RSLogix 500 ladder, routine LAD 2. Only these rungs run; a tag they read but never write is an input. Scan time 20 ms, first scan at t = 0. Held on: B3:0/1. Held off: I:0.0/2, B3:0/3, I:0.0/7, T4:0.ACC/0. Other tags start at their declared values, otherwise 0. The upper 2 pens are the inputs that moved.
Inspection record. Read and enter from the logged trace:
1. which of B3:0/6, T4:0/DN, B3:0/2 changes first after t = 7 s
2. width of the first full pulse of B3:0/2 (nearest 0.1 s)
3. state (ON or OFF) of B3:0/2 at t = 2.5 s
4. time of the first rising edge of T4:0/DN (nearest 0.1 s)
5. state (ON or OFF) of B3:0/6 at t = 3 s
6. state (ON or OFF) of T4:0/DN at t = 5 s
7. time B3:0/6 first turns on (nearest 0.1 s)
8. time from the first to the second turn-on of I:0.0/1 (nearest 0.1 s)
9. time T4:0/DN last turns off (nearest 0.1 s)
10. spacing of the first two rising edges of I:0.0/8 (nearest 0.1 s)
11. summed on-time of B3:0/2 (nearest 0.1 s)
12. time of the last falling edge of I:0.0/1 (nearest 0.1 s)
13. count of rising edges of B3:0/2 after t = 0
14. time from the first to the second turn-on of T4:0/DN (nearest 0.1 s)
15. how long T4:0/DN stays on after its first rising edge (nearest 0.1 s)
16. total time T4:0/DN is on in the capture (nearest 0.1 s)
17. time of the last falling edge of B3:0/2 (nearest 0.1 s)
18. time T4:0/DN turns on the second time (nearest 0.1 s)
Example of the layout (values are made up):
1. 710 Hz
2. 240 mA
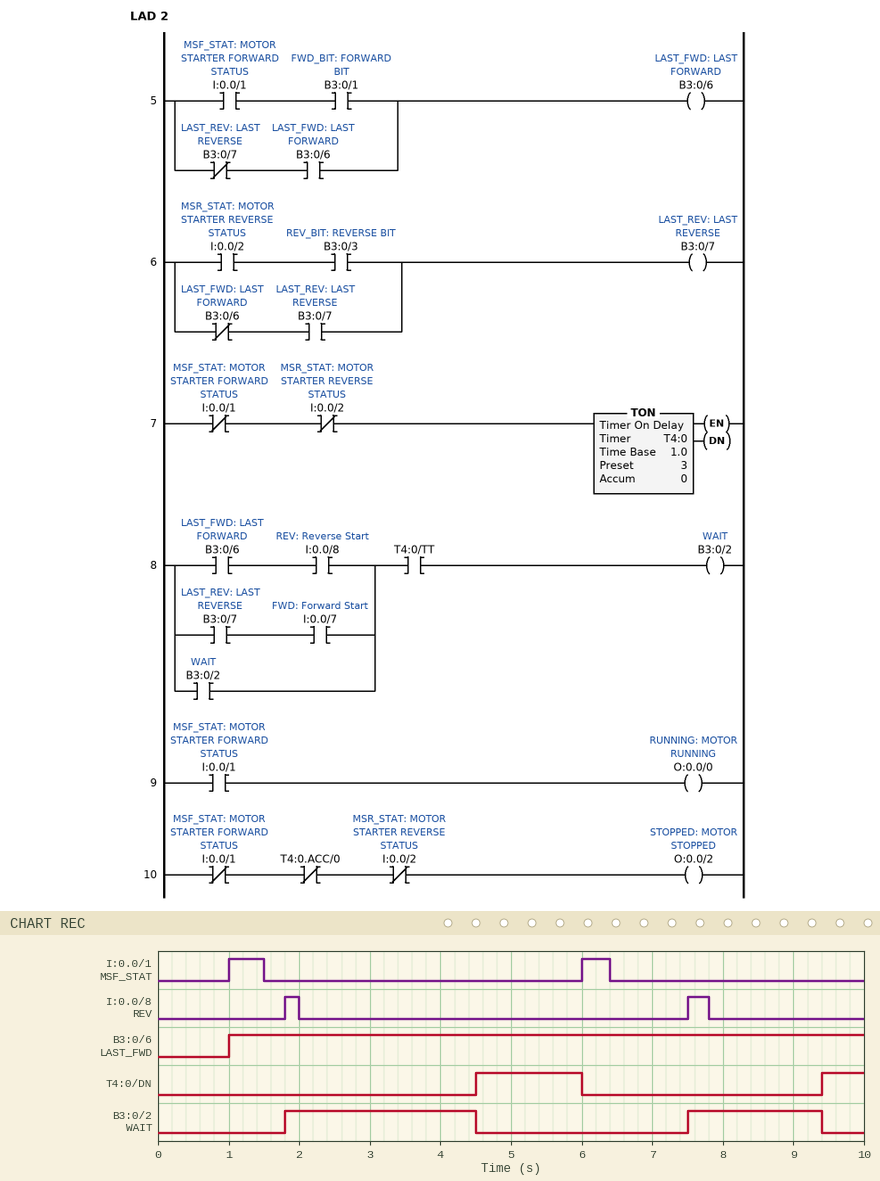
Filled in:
1. B3:0/2
2. 2.7 s
3. ON
4. 4.5 s
5. ON
6. ON
7. 1.0 s
8. 5.0 s
9. 6.0 s
10. 5.7 s
11. 4.6 s
12. 6.4 s
13. 2
14. 4.9 s
15. 1.5 s
16. 2.1 s
17. 9.4 s
18. 9.4 s
